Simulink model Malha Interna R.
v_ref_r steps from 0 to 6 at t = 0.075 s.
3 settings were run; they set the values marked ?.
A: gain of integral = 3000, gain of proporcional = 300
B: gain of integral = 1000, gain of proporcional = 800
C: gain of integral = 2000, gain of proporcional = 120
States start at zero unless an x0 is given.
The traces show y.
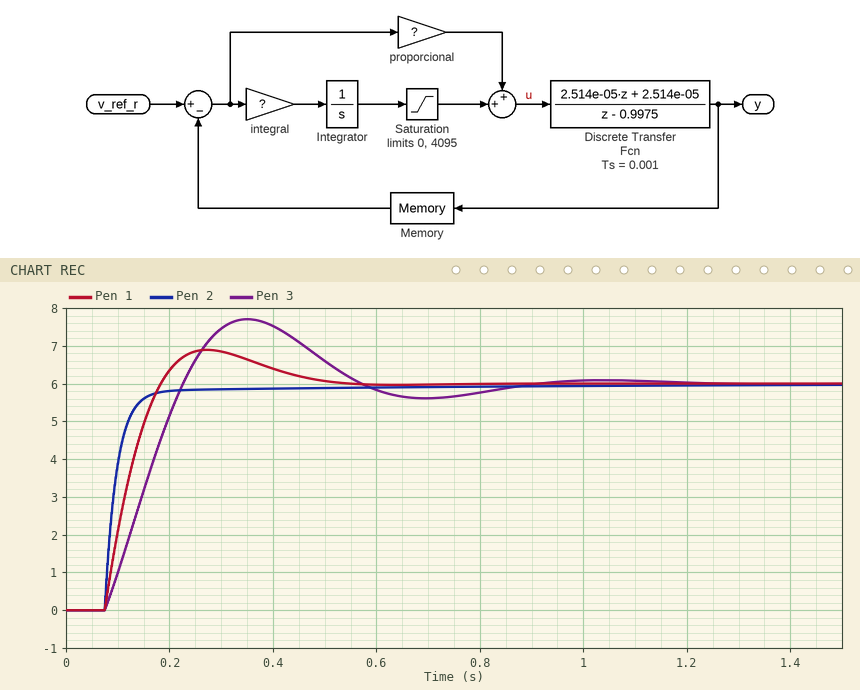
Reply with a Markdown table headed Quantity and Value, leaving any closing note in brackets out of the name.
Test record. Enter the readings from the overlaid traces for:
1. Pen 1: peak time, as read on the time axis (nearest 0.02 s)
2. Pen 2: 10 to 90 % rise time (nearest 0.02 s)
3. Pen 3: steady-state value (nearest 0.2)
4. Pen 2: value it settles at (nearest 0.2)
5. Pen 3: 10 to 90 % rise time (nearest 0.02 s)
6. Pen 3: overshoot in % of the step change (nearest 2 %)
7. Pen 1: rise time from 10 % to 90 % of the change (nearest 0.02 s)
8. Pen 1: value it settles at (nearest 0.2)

| Quantity | Value |
|---|---|
| Pen 1: peak time, as read on the time axis | 0.28 s |
| Pen 2: 10 to 90 % rise time | 0.06 s |
| Pen 3: steady-state value | 6.0 |
| Pen 2: value it settles at | 6.0 |
| Pen 3: 10 to 90 % rise time | 0.12 s |
| Pen 3: overshoot in % of the step change | 28 % |
| Pen 1: rise time from 10 % to 90 % of the change | 0.08 s |
| Pen 1: value it settles at | 6.0 |
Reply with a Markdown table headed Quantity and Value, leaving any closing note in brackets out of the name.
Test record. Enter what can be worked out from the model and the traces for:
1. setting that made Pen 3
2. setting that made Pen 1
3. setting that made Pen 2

| Quantity | Value |
|---|---|
| setting that made Pen 3 | C |
| setting that made Pen 1 | A |
| setting that made Pen 2 | B |
